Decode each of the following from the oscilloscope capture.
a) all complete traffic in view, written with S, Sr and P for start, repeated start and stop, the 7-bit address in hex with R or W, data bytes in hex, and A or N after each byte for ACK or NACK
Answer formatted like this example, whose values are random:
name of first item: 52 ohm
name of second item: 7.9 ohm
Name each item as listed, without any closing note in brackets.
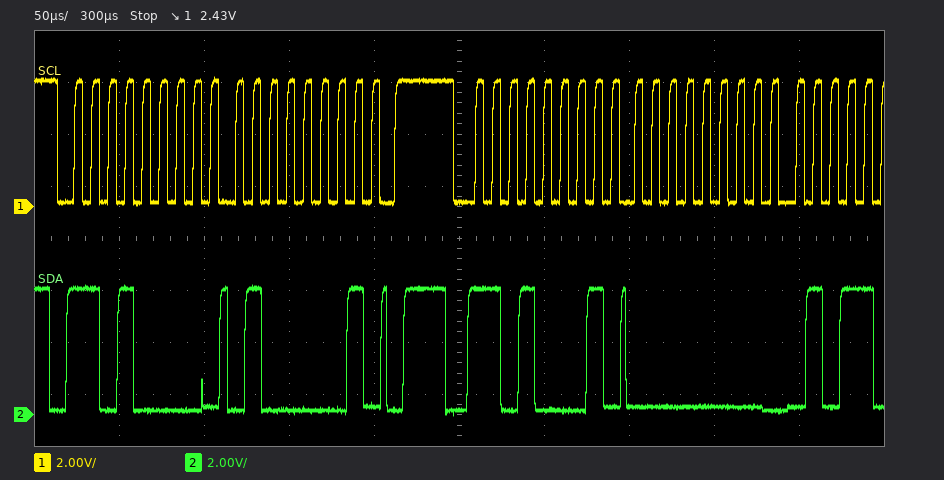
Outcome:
all complete traffic in view, written with S, Sr and P for start, repeated start and stop, the 7-bit address in hex with R or W, data bytes in hex, and A or N after each byte for ACK or NACK: S 68W A 41 A P S 68R A 00 A
